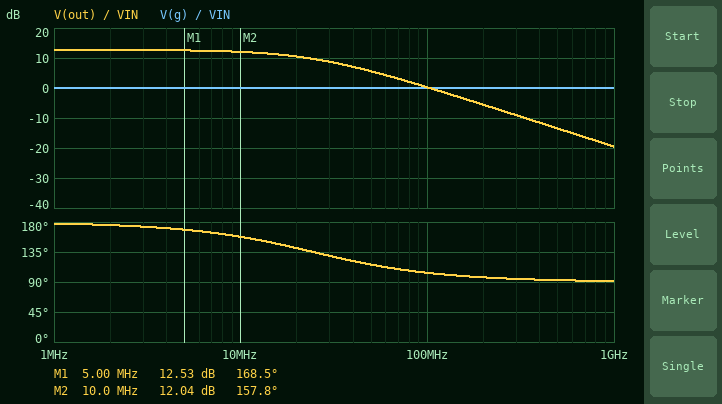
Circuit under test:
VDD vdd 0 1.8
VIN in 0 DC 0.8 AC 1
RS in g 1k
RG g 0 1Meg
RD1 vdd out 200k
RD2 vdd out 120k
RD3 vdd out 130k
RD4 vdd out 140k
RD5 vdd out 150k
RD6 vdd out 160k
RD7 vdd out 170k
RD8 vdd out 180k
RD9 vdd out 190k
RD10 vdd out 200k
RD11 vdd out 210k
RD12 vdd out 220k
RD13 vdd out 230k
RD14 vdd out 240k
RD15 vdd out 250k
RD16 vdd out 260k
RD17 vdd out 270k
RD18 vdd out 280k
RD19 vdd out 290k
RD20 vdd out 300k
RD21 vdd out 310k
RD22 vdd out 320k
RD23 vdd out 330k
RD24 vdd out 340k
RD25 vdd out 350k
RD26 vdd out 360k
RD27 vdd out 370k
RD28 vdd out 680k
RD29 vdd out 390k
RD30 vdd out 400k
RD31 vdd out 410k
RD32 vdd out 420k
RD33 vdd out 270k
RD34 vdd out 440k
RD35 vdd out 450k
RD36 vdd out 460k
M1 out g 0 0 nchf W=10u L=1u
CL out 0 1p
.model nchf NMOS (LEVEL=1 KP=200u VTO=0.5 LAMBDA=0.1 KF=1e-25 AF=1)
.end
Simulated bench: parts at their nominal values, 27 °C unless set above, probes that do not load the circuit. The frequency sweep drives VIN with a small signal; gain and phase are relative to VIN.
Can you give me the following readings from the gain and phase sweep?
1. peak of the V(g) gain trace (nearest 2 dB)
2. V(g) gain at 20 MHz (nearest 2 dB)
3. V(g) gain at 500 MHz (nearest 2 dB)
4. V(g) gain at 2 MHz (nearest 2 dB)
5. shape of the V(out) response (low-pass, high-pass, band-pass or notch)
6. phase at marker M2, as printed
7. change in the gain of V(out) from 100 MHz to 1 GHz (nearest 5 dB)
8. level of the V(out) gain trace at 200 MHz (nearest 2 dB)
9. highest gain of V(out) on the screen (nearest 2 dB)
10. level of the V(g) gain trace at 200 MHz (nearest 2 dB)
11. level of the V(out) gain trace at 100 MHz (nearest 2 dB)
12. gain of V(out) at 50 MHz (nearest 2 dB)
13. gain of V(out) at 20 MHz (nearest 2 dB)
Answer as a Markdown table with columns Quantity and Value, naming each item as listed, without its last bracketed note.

| Quantity | Value |
|---|---|
| peak of the V(g) gain trace | 0 dB |
| V(g) gain at 20 MHz | 0 dB |
| V(g) gain at 500 MHz | 0 dB |
| V(g) gain at 2 MHz | 0 dB |
| shape of the V(out) response | low-pass |
| phase at marker M2, as printed | 157.8 deg |
| change in the gain of V(out) from 100 MHz to 1 GHz | -20 dB |
| level of the V(out) gain trace at 200 MHz | -6 dB |
| highest gain of V(out) on the screen | 12 dB |
| level of the V(g) gain trace at 200 MHz | 0 dB |
| level of the V(out) gain trace at 100 MHz | 0 dB |
| gain of V(out) at 50 MHz | 6 dB |
| gain of V(out) at 20 MHz | 10 dB |
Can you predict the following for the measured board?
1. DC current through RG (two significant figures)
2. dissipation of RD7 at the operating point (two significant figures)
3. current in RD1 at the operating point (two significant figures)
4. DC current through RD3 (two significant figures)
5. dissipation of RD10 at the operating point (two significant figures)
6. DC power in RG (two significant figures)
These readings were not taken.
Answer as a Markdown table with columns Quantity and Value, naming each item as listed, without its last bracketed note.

| Quantity | Value |
|---|---|
| DC current through RG | 800 nA |
| dissipation of RD7 at the operating point | 2.8 µW |
| current in RD1 at the operating point | 3.4 µA |
| DC current through RD3 | 5.3 µA |
| dissipation of RD10 at the operating point | 2.4 µW |
| DC power in RG | 640 nW |
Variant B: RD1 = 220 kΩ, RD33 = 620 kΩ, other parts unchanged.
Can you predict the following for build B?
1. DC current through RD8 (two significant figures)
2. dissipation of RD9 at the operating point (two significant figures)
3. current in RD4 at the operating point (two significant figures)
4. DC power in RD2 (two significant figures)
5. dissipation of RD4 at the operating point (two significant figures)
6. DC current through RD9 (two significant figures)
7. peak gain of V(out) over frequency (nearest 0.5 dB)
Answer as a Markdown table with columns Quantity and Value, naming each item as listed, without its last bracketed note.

| Quantity | Value |
|---|---|
| DC current through RD8 | 3.9 µA |
| dissipation of RD9 at the operating point | 2.6 µW |
| current in RD4 at the operating point | 5.0 µA |
| DC power in RD2 | 4.1 µW |
| dissipation of RD4 at the operating point | 3.5 µW |
| DC current through RD9 | 3.7 µA |
| peak gain of V(out) over frequency | 13.0 dB |
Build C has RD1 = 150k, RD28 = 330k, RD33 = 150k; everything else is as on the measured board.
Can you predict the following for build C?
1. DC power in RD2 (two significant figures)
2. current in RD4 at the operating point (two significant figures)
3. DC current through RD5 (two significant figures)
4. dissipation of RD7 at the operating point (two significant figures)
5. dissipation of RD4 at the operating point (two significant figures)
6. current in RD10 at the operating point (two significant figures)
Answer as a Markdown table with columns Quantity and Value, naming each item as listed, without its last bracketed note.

| Quantity | Value |
|---|---|
| DC power in RD2 | 3.6 µW |
| current in RD4 at the operating point | 4.7 µA |
| DC current through RD5 | 4.4 µA |
| dissipation of RD7 at the operating point | 2.6 µW |
| dissipation of RD4 at the operating point | 3.1 µW |
| current in RD10 at the operating point | 3.3 µA |
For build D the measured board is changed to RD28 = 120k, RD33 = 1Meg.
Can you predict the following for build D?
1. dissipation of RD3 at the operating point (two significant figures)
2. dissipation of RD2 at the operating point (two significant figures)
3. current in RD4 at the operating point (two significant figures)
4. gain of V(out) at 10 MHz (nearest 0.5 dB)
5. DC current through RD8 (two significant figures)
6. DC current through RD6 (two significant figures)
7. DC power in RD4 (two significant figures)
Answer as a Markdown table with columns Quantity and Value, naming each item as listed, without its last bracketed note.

| Quantity | Value |
|---|---|
| dissipation of RD3 at the operating point | 3.4 µW |
| dissipation of RD2 at the operating point | 3.7 µW |
| current in RD4 at the operating point | 4.8 µA |
| gain of V(out) at 10 MHz | 12.0 dB |
| DC current through RD8 | 3.7 µA |
| DC current through RD6 | 4.2 µA |
| DC power in RD4 | 3.2 µW |
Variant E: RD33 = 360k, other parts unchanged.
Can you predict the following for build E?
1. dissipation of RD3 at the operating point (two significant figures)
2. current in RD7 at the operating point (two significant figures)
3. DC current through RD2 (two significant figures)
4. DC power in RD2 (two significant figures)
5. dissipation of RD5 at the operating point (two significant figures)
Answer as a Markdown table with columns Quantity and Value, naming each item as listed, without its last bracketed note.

| Quantity | Value |
|---|---|
| dissipation of RD3 at the operating point | 3.7 µW |
| current in RD7 at the operating point | 4.1 µA |
| DC current through RD2 | 5.8 µA |
| DC power in RD2 | 4.0 µW |
| dissipation of RD5 at the operating point | 3.2 µW |
